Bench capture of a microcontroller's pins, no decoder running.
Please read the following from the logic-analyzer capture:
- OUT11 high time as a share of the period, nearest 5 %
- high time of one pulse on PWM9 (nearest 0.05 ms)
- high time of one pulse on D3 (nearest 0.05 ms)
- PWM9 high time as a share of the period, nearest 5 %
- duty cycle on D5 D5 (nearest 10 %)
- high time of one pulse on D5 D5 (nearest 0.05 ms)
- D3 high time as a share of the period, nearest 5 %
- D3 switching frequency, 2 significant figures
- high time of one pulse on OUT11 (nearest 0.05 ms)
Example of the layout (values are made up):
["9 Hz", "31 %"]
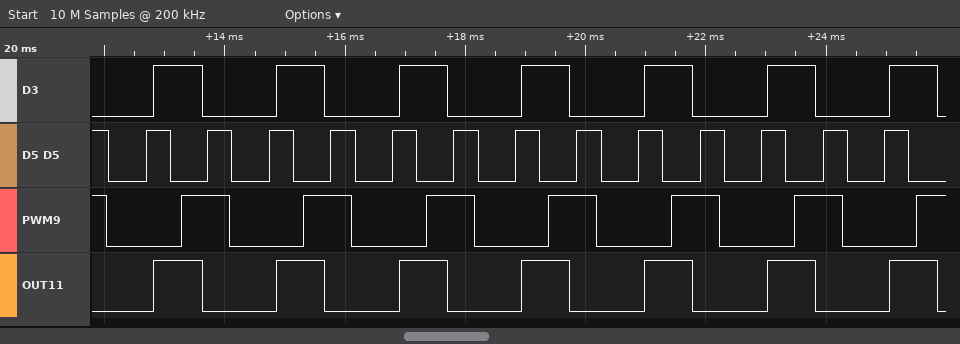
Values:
["40 %", "0.80 ms", "0.80 ms", "40 %", "40 %", "0.40 ms", "40 %", "490 Hz", "0.80 ms"]
